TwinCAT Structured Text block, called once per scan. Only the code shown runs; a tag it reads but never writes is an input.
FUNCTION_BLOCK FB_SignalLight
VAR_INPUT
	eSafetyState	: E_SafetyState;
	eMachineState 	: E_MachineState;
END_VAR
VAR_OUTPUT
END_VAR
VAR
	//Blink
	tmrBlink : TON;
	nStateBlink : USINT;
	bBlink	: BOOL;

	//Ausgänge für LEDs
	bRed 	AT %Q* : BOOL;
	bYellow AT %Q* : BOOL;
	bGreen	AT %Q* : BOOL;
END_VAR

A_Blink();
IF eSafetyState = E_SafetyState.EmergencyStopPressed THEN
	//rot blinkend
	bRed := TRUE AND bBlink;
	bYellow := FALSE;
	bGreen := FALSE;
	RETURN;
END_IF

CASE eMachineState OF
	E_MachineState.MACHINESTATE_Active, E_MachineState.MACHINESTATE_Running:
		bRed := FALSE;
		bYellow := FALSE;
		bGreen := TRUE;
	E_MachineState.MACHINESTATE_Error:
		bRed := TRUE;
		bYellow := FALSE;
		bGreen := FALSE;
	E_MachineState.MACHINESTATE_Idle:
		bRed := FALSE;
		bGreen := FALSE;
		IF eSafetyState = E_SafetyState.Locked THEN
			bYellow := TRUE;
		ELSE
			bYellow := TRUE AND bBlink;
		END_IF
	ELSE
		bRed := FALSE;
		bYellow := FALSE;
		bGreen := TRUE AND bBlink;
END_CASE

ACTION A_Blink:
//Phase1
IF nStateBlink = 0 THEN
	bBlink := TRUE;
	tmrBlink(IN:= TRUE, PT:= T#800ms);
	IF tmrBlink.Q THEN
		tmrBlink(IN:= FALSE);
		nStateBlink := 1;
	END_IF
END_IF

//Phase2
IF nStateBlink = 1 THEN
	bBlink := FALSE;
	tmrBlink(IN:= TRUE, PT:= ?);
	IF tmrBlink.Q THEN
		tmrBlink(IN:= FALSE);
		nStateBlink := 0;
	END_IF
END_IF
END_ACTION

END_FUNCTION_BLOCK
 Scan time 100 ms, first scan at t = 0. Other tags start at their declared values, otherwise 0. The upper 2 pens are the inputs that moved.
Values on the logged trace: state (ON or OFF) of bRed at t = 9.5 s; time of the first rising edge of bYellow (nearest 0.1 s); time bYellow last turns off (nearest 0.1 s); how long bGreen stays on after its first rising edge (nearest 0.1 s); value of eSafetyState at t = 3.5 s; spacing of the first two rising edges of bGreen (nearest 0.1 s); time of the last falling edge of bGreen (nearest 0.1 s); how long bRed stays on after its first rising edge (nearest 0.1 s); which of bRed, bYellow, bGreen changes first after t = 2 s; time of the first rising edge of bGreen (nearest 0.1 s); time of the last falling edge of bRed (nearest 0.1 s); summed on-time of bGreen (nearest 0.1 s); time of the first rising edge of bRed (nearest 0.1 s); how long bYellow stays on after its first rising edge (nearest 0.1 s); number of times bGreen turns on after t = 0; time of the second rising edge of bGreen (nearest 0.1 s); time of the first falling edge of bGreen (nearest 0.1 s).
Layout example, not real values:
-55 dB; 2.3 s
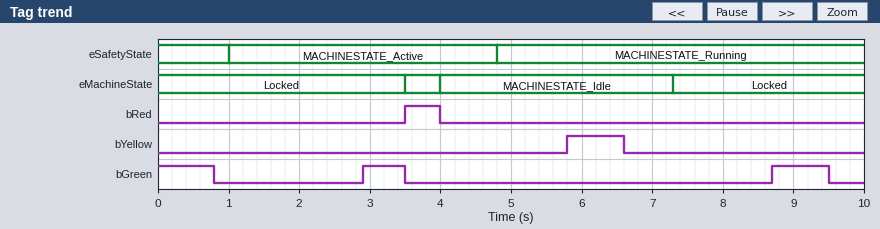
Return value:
OFF; 5.8 s; 6.6 s; 0.6 s; MACHINESTATE_Active; 5.8 s; 9.5 s; 0.5 s; bGreen; 2.9 s; 4.0 s; 2.2 s; 3.5 s; 0.8 s; 2; 8.7 s; 0.8 s
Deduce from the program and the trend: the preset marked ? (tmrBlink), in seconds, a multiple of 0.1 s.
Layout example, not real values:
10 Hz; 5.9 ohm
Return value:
2.0 s
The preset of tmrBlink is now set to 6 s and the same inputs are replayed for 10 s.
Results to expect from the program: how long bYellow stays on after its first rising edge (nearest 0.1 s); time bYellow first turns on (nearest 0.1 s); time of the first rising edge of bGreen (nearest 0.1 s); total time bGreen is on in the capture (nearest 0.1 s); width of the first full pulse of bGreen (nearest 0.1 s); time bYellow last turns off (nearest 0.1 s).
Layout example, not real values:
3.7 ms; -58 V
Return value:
0.4 s; 6.9 s; 7.3 s; 1.2 s; 0.4 s; 7.3 s
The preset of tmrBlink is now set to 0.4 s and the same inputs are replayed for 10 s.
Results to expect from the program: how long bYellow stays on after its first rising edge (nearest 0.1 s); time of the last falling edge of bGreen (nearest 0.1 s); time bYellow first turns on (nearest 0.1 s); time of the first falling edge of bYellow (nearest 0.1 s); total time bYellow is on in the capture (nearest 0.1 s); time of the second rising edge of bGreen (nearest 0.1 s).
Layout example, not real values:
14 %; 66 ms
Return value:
0.7 s; 9.9 s; 4.0 s; 4.7 s; 2.3 s; 2.6 s
